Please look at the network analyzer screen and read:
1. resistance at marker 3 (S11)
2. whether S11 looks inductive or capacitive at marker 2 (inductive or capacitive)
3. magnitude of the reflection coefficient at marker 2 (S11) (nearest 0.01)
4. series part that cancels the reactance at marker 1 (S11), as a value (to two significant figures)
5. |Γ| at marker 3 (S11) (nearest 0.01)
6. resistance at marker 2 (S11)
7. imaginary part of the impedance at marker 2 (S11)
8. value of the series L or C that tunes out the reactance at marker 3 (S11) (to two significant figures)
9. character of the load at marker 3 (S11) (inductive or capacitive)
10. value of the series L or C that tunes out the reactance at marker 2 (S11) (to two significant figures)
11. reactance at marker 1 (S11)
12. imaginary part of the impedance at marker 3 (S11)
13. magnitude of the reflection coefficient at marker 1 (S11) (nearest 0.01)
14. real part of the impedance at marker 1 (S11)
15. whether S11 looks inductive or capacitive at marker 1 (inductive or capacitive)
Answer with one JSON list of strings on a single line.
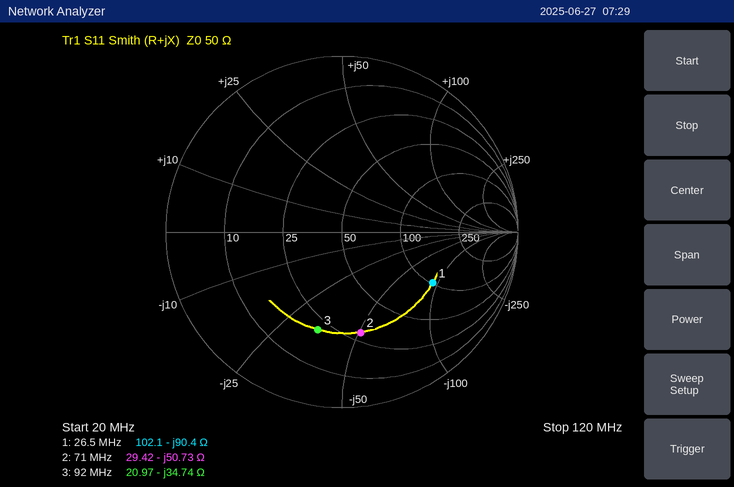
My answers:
["20.97 Ω", "capacitive", "0.58", "540 nH", "0.57", "29.42 Ω", "-50.73 Ω", "60 nH", "capacitive", "110 nH", "-90.4 Ω", "-34.74 Ω", "0.59", "102.1 Ω", "capacitive"]
